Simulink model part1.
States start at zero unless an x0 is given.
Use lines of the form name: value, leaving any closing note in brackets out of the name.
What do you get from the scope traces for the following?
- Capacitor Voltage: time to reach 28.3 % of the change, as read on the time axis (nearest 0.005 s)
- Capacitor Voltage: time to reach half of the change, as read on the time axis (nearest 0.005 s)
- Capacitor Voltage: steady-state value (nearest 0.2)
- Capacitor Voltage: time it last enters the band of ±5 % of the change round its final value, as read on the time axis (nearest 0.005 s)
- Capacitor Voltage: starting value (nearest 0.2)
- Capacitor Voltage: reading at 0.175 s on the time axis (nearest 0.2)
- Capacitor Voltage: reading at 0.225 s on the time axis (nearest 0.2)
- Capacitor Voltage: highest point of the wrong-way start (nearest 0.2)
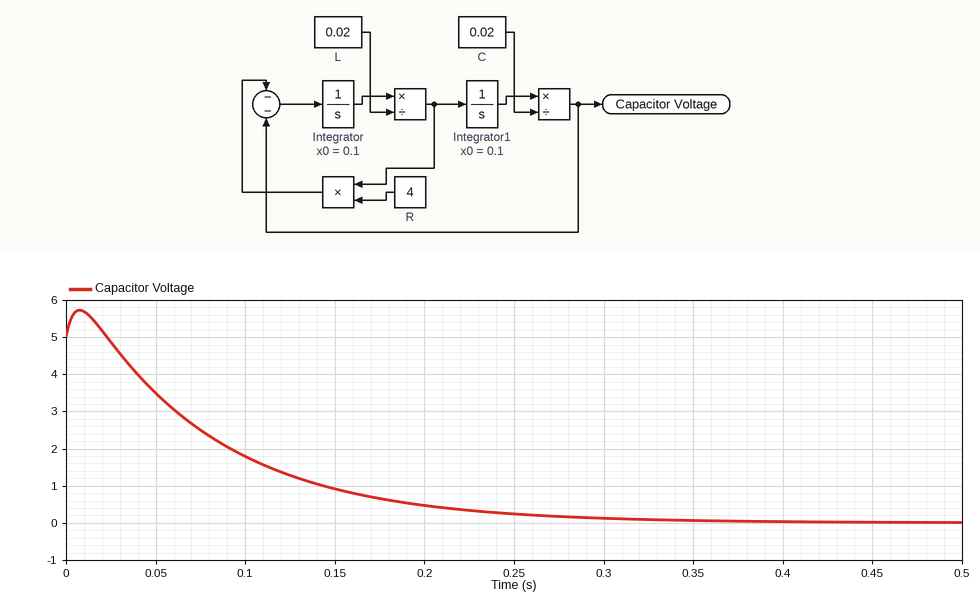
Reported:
Capacitor Voltage: time to reach 28.3 % of the change, as read on the time axis: 0.050 s
Capacitor Voltage: time to reach half of the change, as read on the time axis: 0.075 s
Capacitor Voltage: steady-state value: 0.0
Capacitor Voltage: time it last enters the band of ±5 % of the change round its final value, as read on the time axis: 0.245 s
Capacitor Voltage: starting value: 5.0
Capacitor Voltage: reading at 0.175 s on the time axis: 0.6
Capacitor Voltage: reading at 0.225 s on the time axis: 0.4
Capacitor Voltage: highest point of the wrong-way start: 5.8
